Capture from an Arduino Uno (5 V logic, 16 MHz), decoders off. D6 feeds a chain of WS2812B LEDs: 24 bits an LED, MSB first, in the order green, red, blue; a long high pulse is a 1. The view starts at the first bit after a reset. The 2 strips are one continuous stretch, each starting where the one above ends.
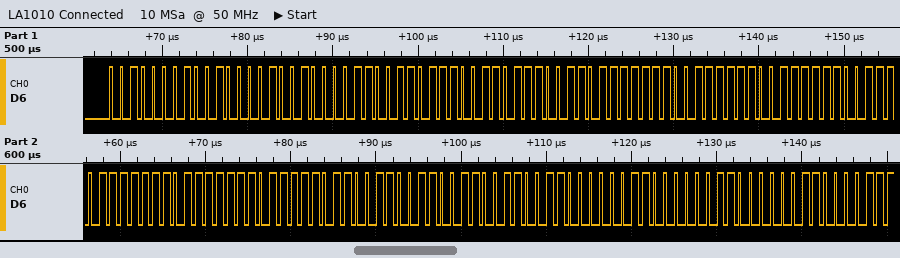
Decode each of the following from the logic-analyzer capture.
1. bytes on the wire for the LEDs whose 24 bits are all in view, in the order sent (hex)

21 21 21 9B 9B 9B F9 F9 F9 DF DF DF 66 66 66 06 06 06
